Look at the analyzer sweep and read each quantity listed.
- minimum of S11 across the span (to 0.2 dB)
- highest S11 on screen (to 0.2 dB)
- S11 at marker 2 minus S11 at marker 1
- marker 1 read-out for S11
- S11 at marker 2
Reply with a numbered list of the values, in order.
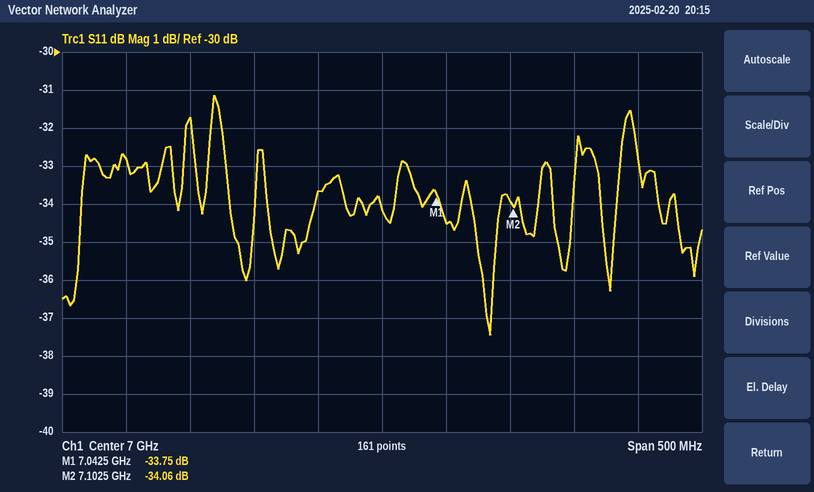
1. -37.4 dB
2. -31.2 dB
3. -0.31 dB
4. -33.75 dB
5. -34.06 dB
